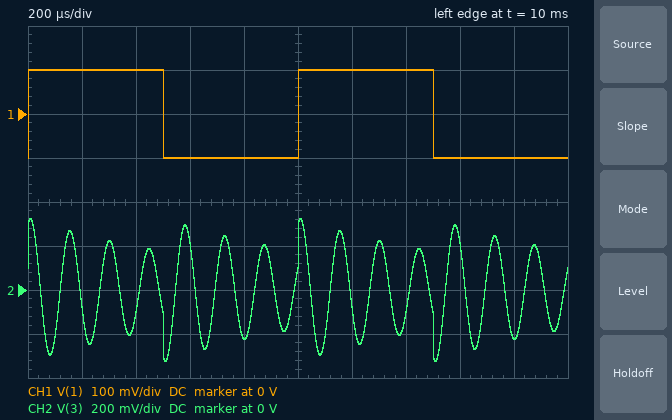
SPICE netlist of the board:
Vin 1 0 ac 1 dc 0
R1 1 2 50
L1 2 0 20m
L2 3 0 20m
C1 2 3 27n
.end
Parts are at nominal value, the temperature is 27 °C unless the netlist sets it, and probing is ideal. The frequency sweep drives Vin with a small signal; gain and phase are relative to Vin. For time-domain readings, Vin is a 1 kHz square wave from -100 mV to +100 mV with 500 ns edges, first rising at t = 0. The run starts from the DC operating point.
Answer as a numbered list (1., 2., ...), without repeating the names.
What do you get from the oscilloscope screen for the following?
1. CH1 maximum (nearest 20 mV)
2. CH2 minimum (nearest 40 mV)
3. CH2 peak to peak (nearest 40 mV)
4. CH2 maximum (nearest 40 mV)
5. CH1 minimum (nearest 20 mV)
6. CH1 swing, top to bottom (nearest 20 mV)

1. 100 mV
2. -320 mV
3. 640 mV
4. 320 mV
5. -100 mV
6. 200 mV
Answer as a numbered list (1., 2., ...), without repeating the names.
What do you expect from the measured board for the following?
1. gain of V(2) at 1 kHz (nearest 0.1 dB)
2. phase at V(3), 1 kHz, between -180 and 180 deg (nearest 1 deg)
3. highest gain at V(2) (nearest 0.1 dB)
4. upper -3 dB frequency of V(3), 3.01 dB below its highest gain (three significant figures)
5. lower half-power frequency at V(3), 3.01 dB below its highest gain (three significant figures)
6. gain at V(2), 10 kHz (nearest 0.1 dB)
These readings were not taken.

1. -0.6 dB
2. -159 deg
3. 0 dB
4. 7.05 kHz
5. 6.65 kHz
6. -0.1 dB
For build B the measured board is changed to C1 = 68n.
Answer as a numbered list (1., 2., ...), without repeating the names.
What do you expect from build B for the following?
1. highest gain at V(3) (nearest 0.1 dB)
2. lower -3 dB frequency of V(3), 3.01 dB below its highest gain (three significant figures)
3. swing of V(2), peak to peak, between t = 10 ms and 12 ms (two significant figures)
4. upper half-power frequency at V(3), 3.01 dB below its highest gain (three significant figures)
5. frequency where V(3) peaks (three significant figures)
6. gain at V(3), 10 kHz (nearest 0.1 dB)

1. 20.7 dB
2. 4.12 kHz
3. 320 mV
4. 4.52 kHz
5. 4.31 kHz
6. 1.8 dB
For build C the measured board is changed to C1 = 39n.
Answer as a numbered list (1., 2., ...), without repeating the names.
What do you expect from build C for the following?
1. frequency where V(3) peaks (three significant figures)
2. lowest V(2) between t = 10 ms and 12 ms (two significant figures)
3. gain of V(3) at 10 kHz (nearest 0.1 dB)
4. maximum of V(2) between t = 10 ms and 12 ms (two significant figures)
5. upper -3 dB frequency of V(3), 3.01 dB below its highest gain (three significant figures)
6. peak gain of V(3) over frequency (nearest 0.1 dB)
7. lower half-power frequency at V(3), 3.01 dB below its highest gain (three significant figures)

1. 5.69 kHz
2. -150 mV
3. 3.4 dB
4. 150 mV
5. 5.90 kHz
6. 23.1 dB
7. 5.50 kHz
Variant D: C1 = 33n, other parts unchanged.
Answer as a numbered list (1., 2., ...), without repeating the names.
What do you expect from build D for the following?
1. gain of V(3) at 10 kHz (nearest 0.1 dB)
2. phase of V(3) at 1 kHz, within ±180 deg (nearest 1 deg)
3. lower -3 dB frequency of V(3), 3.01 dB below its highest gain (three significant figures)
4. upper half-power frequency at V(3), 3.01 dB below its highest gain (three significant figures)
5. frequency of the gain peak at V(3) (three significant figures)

1. 4.2 dB
2. -159 deg
3. 6.00 kHz
4. 6.40 kHz
5. 6.19 kHz
